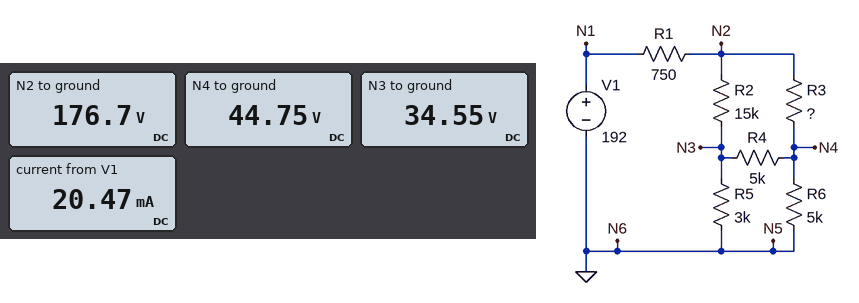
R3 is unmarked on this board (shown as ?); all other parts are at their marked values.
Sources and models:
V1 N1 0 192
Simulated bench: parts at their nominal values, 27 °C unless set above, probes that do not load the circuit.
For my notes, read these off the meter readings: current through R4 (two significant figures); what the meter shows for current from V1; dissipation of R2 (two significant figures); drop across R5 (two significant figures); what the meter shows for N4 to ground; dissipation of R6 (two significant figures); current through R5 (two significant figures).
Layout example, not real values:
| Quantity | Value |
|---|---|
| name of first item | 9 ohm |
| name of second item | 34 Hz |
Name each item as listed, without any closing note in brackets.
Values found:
| Quantity | Value |
|---|---|
| current through R4 | 2.0 mA |
| what the meter shows for current from V1 | 20.47 mA |
| dissipation of R2 | 1.3 W |
| drop across R5 | 35 V |
| what the meter shows for N4 to ground | 44.75 V |
| dissipation of R6 | 400 mW |
| current through R5 | 12 mA |
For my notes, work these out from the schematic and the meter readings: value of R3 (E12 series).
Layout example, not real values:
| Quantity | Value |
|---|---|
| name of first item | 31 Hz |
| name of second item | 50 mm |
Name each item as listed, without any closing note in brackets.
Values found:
| Quantity | Value |
|---|---|
| value of R3 | 12 kΩ |
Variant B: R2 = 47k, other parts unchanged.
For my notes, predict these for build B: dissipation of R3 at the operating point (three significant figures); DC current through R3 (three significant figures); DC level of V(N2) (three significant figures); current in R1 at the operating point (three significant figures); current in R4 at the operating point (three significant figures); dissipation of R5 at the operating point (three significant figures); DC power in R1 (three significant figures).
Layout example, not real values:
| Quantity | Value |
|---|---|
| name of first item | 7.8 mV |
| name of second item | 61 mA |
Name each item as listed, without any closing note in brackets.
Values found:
| Quantity | Value |
|---|---|
| dissipation of R3 at the operating point | 1.65 W |
| DC current through R3 | 11.7 mA |
| DC level of V(N2) | 181 V |
| current in R1 at the operating point | 15.1 mA |
| current in R4 at the operating point | 3.73 mA |
| dissipation of R5 at the operating point | 152 mW |
| DC power in R1 | 171 mW |
